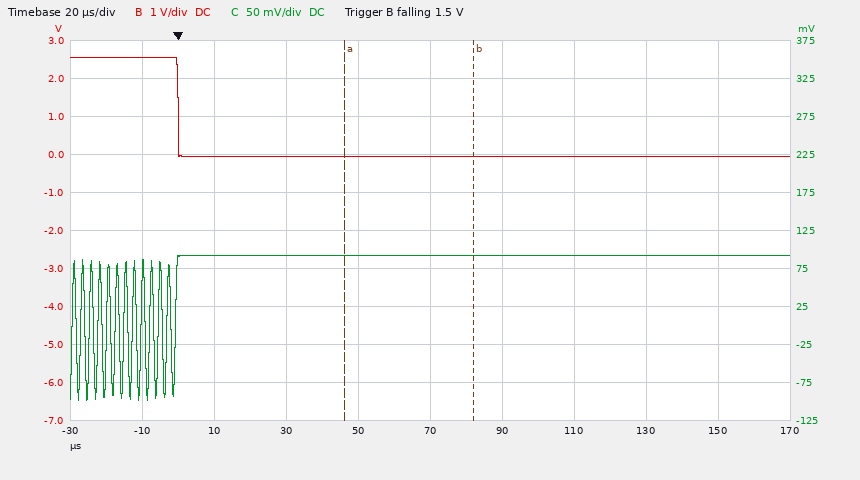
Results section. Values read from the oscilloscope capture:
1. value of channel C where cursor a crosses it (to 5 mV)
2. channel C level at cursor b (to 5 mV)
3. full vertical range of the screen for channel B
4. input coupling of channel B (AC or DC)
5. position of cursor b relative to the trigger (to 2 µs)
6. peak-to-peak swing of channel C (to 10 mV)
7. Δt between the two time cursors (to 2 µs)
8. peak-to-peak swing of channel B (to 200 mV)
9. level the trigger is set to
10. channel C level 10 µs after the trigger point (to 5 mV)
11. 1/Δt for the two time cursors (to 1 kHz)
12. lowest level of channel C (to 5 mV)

90 mV
90 mV
10 V
DC
+82 µs
190 mV
36 µs
2.6 V
1.5 V
90 mV
28 kHz
-100 mV
